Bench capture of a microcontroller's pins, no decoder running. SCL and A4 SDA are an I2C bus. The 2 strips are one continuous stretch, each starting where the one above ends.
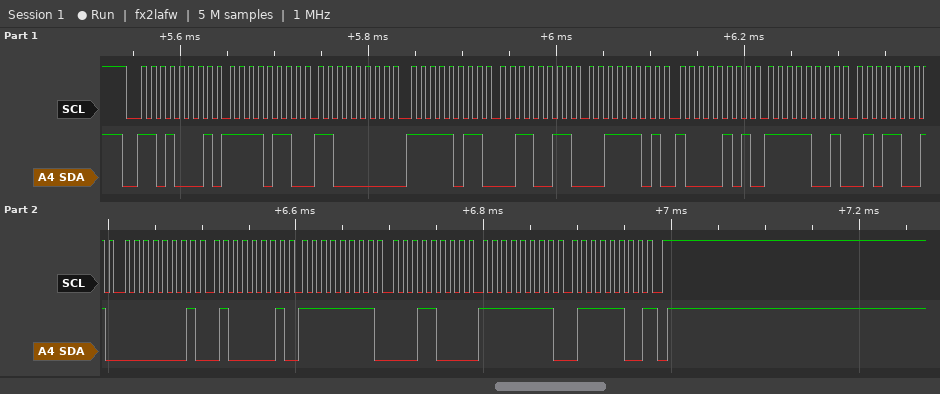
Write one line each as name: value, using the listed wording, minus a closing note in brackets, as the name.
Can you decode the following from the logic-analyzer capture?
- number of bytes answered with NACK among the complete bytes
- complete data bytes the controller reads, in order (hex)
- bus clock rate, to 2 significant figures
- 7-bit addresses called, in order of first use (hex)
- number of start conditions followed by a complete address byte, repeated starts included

number of bytes answered with NACK among the complete bytes: 1
complete data bytes the controller reads, in order: F6 C0 FB 33 3D 85 F9 59 01 41 FF 18 FF 7C
bus clock rate, to 2 significant figures: 100 kHz
7-bit addresses called, in order of first use: 0x68
number of start conditions followed by a complete address byte, repeated starts included: 1
